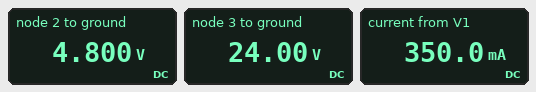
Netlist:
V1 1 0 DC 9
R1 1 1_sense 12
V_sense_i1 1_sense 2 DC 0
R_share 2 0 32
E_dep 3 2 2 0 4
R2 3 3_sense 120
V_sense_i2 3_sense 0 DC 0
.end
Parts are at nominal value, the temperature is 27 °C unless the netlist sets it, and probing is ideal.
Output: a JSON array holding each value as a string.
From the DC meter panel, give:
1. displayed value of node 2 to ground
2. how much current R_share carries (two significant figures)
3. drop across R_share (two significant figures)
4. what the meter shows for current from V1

["4.800 V", "150 mA", "4.8 V", "350.0 mA"]
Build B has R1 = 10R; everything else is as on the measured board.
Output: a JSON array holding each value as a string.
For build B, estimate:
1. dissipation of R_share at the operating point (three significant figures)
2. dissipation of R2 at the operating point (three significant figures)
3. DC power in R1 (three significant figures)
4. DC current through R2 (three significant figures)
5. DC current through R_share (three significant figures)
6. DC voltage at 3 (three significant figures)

["847 mW", "5.64 W", "1.44 W", "217 mA", "163 mA", "26.0 V"]
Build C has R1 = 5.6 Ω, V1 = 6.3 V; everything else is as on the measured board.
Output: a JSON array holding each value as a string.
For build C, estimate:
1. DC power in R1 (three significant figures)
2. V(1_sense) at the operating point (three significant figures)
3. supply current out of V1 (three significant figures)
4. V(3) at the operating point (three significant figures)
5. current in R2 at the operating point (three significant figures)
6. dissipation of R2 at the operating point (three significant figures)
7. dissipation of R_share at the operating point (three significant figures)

["596 mW", "4.47 V", "326 mA", "22.4 V", "186 mA", "4.17 W", "625 mW"]
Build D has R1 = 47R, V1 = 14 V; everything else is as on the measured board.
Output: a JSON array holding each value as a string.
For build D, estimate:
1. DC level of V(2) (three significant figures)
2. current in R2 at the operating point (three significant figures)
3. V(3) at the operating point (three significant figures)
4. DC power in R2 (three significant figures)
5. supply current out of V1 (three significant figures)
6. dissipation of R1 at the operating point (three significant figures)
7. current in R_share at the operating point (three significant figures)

["3.16 V", "132 mA", "15.8 V", "2.08 W", "231 mA", "2.50 W", "98.8 mA"]
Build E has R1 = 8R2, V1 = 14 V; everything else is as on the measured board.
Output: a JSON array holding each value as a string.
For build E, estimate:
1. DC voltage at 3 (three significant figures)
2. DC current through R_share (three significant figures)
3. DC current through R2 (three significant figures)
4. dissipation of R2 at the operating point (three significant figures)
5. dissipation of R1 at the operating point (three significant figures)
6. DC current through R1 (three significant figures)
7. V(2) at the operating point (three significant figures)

["43.8 V", "274 mA", "365 mA", "16.0 W", "3.35 W", "639 mA", "8.76 V"]
